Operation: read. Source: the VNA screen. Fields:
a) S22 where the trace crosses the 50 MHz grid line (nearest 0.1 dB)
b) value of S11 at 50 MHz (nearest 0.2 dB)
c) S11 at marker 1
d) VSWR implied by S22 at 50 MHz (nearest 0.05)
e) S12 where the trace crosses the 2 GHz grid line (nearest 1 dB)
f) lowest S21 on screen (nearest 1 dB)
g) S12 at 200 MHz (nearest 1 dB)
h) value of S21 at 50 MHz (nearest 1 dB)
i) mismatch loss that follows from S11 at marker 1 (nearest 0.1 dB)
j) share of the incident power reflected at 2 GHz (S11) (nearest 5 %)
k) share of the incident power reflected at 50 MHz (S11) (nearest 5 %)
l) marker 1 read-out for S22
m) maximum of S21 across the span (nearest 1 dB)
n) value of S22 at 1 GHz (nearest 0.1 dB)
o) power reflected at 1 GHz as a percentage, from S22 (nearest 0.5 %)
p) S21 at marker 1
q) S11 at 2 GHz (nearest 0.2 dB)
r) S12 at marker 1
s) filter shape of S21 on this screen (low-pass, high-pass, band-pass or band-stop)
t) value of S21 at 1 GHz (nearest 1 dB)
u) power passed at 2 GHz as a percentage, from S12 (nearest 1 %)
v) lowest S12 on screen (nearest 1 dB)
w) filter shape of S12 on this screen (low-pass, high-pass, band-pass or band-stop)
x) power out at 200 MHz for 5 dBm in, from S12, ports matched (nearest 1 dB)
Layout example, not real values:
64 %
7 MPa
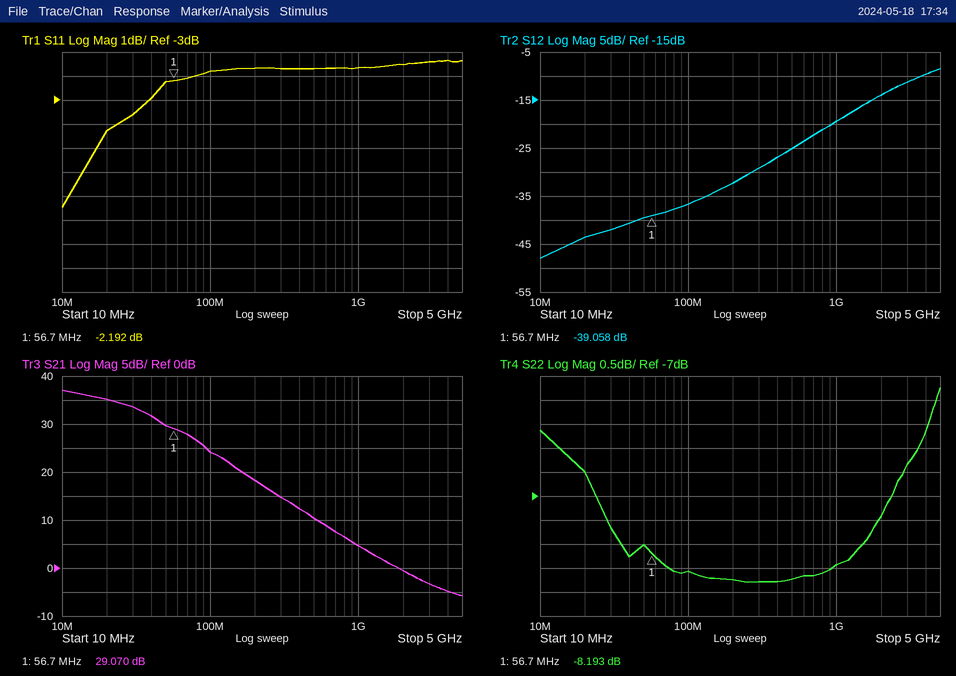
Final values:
-8.0 dB
-2.2 dB
-2.192 dB
2.30
-14 dB
-6 dB
-32 dB
30 dB
4.0 dB
70 %
60 %
-8.193 dB
37 dB
-8.4 dB
14.5 %
29.070 dB
-1.6 dB
-39.058 dB
low-pass
5 dB
4 %
-48 dB
high-pass
-27 dBm
